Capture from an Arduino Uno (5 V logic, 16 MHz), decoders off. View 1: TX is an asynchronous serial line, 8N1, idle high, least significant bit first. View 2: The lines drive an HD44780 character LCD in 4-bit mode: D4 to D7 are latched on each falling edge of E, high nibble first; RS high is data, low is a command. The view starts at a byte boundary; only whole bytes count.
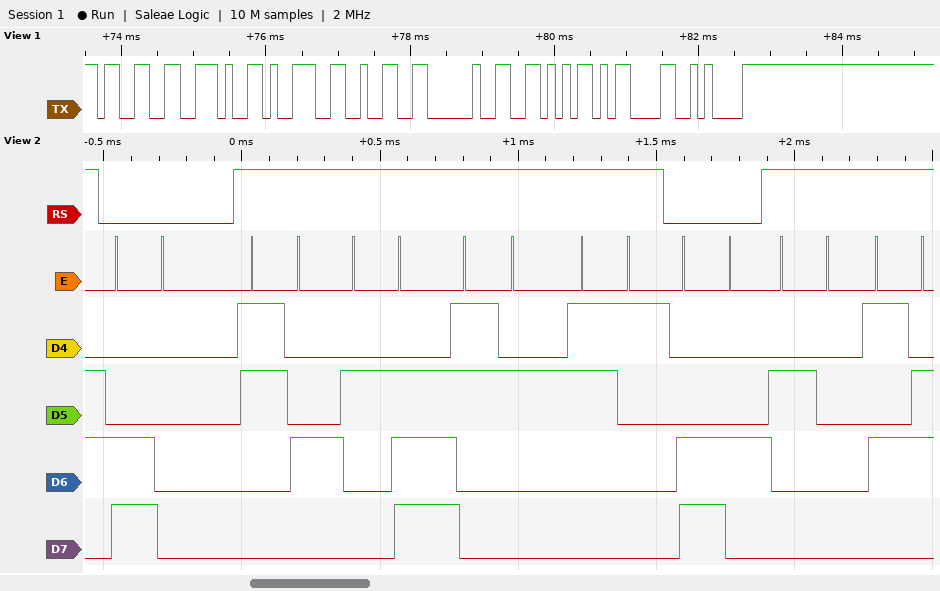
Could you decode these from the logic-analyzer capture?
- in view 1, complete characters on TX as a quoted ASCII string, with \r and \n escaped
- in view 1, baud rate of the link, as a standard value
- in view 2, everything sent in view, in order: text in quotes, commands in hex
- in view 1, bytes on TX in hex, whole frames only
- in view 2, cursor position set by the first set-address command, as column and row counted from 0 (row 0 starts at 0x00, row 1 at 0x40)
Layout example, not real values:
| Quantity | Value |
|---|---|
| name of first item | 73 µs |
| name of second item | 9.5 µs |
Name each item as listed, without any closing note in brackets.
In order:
| Quantity | Value |
|---|---|
| in view 1, complete characters on TX as a quoted ASCII string, with \r and \n escaped | "3.92 V\r\n" |
| in view 1, baud rate of the link, as a standard value | 9600 baud |
| in view 2, everything sent in view, in order: text in quotes, commands in hex | 0xC0 "4.21" 0xC4 " V" |
| in view 1, bytes on TX in hex, whole frames only | 33 2E 39 32 20 56 0D 0A |
| in view 2, cursor position set by the first set-address command, as column and row counted from 0 | column 0, row 1 |
